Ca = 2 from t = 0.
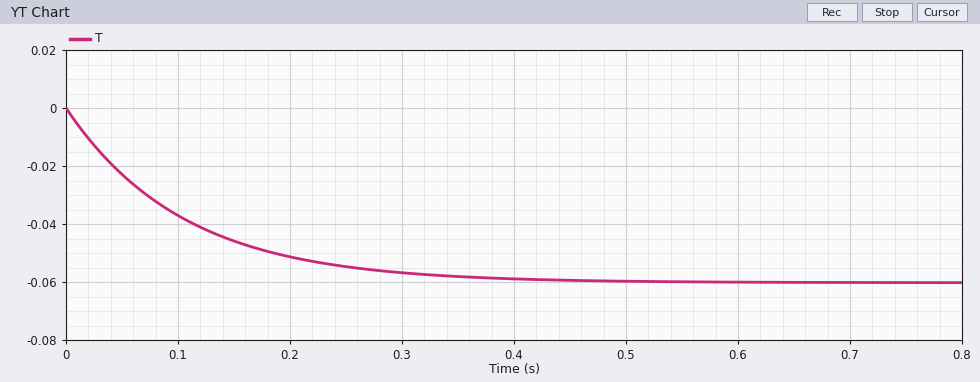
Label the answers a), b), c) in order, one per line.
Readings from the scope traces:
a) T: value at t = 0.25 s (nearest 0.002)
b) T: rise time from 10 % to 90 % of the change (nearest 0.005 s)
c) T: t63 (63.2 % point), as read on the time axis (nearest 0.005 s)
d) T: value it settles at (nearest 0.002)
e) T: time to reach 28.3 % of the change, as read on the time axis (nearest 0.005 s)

a) -0.054
b) 0.230 s
c) 0.105 s
d) -0.060
e) 0.035 s
